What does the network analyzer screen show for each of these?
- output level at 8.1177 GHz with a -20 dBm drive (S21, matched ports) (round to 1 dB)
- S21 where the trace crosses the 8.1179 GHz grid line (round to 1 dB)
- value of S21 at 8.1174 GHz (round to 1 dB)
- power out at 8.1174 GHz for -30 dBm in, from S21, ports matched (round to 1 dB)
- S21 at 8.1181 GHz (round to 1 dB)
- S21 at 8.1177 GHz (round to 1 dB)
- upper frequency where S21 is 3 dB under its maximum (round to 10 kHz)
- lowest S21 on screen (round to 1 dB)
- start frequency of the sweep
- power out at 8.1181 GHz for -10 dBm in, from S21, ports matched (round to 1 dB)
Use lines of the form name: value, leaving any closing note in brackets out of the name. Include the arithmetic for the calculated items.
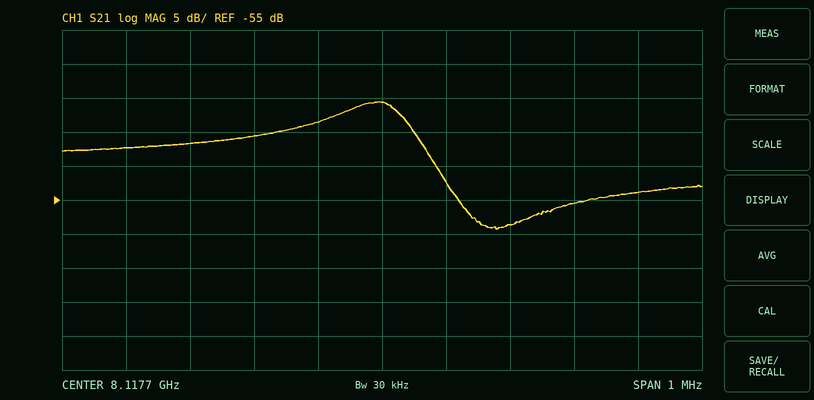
output level at 8.1177 GHz with a -20 dBm drive (S21, matched ports): -20 dBm + (-41 dB) = -61 dBm
S21 where the trace crosses the 8.1179 GHz grid line: -59 dB
value of S21 at 8.1174 GHz: -47 dB
power out at 8.1174 GHz for -30 dBm in, from S21, ports matched: -30 dBm + (-47 dB) = -77 dBm
S21 at 8.1181 GHz: -54 dB
S21 at 8.1177 GHz: -41 dB
upper frequency where S21 is 3 dB under its maximum: 8.11774 GHz
lowest S21 on screen: -59 dB
start frequency of the sweep: 8.1172 GHz
power out at 8.1181 GHz for -10 dBm in, from S21, ports matched: -10 dBm + (-54 dB) = -64 dBm
